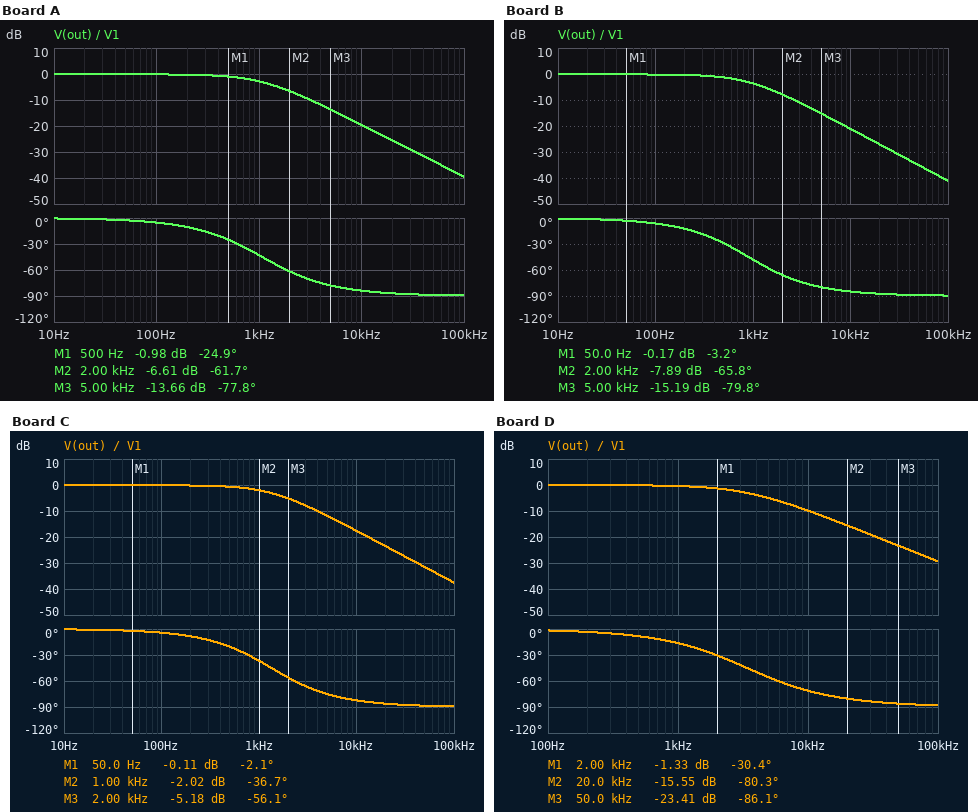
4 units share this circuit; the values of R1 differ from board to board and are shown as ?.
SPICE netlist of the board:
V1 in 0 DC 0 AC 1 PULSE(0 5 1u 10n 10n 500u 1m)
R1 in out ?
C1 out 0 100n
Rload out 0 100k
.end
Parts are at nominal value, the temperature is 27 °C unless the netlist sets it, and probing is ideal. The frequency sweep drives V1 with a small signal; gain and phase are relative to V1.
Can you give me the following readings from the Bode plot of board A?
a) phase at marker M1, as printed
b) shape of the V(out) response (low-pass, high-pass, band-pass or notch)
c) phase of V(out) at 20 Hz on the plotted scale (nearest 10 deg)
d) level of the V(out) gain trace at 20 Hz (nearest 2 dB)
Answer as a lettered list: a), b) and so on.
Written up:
a) -24.9 deg
b) low-pass
c) 0 deg
d) 0 dB
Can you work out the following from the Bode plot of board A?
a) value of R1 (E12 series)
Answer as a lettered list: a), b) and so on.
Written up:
a) 1.5 kΩ
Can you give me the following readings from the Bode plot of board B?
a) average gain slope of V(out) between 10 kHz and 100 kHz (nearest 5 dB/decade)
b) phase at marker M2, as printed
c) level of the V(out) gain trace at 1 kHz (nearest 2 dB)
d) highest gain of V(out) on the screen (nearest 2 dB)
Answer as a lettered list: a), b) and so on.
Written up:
a) -20 dB/decade
b) -65.8 deg
c) -4 dB
d) 0 dB
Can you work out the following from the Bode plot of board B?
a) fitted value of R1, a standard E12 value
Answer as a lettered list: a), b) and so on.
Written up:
a) 1.8 kΩ
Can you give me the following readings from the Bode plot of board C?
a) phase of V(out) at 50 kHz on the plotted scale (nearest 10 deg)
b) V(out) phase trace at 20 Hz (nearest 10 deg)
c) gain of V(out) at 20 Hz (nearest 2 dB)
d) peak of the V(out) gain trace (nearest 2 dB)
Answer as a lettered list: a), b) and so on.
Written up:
a) -90 deg
b) 0 deg
c) 0 dB
d) 0 dB
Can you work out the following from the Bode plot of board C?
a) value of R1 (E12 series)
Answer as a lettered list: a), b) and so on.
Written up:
a) 1.2 kΩ
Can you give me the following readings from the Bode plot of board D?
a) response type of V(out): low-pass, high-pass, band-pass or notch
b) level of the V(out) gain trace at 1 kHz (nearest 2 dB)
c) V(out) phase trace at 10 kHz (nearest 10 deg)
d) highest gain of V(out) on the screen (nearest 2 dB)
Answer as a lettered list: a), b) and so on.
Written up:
a) low-pass
b) 0 dB
c) -70 deg
d) 0 dB
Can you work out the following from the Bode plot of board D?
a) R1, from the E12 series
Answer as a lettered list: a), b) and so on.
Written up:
a) 470 Ω
